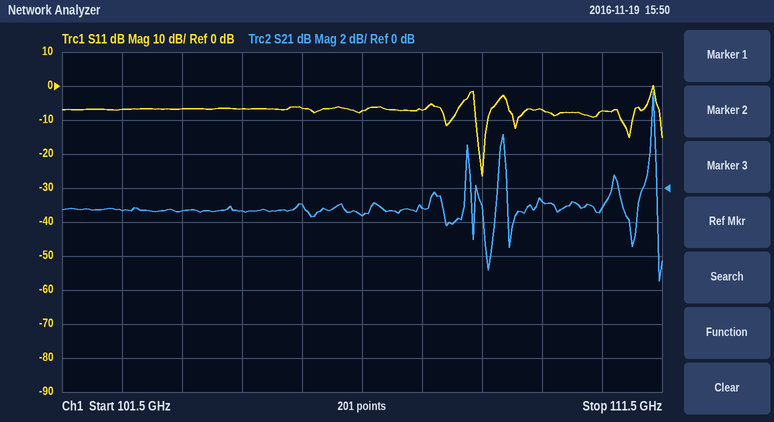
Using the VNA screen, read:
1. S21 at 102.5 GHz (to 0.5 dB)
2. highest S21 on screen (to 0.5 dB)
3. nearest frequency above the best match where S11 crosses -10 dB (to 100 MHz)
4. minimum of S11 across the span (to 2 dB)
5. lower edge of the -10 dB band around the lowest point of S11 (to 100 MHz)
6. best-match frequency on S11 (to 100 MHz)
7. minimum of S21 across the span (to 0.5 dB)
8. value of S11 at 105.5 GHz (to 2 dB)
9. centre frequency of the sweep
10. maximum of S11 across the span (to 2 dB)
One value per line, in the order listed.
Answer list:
-1.5 dB
5.5 dB
108.6 GHz
-26 dB
108.4 GHz
108.5 GHz
-5.5 dB
-6 dB
106.5 GHz
0 dB
